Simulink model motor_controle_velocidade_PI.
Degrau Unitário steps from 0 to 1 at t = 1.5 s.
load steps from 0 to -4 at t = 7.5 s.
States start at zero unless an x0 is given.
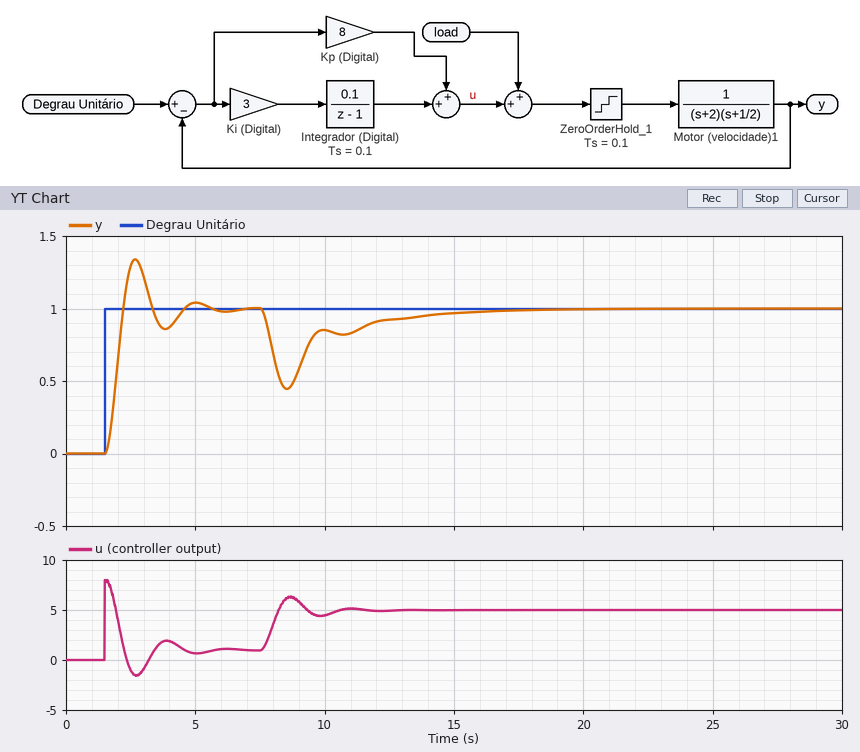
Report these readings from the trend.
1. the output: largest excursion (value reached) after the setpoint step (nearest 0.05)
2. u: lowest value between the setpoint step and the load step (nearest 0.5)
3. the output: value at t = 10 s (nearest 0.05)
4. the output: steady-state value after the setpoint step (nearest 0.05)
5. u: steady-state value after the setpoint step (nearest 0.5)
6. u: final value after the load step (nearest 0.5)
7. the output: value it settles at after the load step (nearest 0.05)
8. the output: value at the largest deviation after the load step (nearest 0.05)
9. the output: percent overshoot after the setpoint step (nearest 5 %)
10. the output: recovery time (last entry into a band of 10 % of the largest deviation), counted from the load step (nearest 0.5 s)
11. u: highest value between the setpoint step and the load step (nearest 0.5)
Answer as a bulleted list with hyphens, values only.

- 1.35
- -1.5
- 0.85
- 1.00
- 1.0
- 5.0
- 1.00
- 0.45
- 35 %
- 6.0 s
- 8.0
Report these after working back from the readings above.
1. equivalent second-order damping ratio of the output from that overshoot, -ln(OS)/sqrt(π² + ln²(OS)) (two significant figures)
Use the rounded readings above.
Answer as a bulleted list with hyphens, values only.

- 0.32
